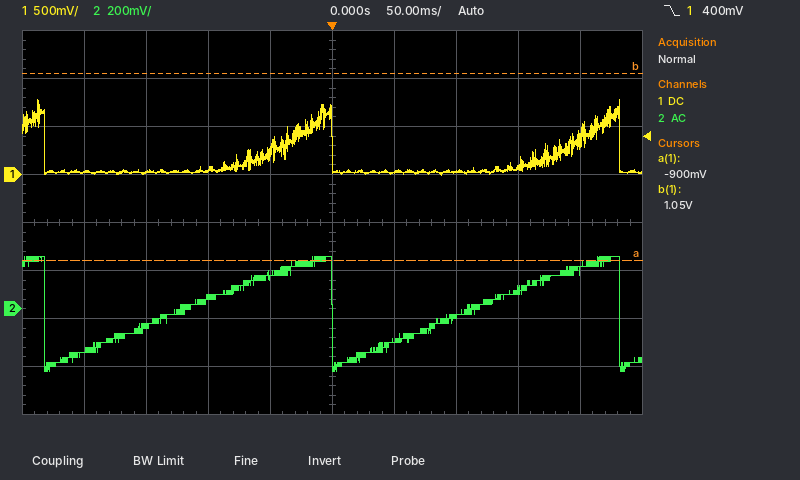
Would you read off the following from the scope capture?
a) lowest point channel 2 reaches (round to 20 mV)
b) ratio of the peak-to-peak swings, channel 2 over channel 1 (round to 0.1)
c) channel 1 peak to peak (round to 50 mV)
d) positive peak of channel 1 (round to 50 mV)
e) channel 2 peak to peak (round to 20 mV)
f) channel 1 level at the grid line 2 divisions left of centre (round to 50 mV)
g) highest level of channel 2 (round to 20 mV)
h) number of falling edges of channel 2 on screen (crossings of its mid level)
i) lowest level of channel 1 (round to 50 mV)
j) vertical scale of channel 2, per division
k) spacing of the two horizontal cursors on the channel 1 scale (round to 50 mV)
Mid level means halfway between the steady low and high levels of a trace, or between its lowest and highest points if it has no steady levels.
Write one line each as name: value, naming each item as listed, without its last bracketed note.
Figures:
lowest point channel 2 reaches: -260 mV
ratio of the peak-to-peak swings, channel 2 over channel 1: 0.6
channel 1 peak to peak: 800 mV
positive peak of channel 1: 800 mV
channel 2 peak to peak: 480 mV
channel 1 level at the grid line 2 divisions left of centre: 50 mV
highest level of channel 2: 220 mV
number of falling edges of channel 2 on screen: 3
lowest level of channel 1: 0 mV
vertical scale of channel 2, per division: 200 mV
spacing of the two horizontal cursors on the channel 1 scale: 1.95 V
